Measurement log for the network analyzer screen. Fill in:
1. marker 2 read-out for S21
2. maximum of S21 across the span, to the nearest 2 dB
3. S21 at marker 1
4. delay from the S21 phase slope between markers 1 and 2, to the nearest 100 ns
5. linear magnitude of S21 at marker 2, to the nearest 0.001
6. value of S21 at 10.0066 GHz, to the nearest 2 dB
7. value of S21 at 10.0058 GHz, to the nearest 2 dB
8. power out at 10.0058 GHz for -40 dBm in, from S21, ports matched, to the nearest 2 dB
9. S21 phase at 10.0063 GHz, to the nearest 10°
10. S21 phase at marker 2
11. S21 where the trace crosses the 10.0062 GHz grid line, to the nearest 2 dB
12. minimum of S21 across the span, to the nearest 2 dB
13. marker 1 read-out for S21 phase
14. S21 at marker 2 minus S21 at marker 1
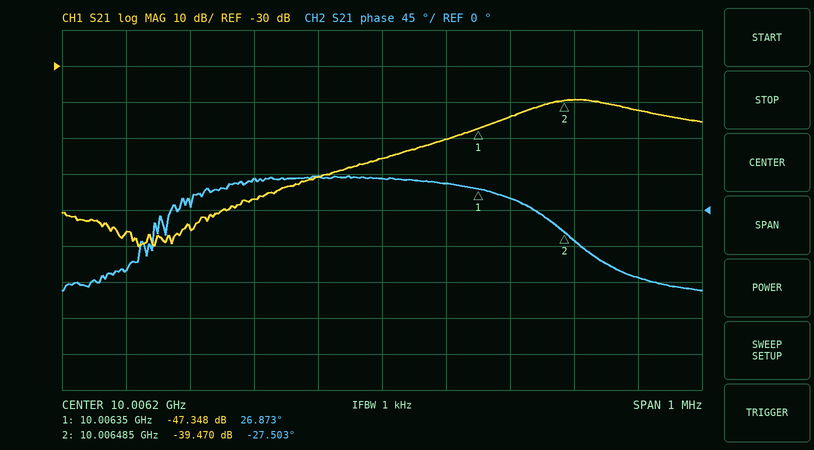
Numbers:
-39.470 dB
-40 dB
-47.348 dB
1.1 µs
0.011
-42 dB
-76 dB
-116 dBm
30°
-27.503°
-56 dB
-80 dB
26.873°
7.878 dB
